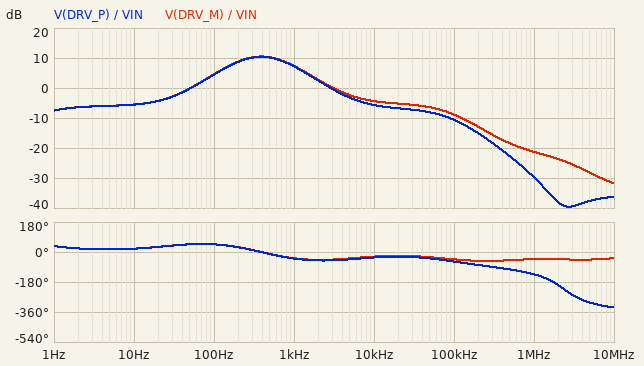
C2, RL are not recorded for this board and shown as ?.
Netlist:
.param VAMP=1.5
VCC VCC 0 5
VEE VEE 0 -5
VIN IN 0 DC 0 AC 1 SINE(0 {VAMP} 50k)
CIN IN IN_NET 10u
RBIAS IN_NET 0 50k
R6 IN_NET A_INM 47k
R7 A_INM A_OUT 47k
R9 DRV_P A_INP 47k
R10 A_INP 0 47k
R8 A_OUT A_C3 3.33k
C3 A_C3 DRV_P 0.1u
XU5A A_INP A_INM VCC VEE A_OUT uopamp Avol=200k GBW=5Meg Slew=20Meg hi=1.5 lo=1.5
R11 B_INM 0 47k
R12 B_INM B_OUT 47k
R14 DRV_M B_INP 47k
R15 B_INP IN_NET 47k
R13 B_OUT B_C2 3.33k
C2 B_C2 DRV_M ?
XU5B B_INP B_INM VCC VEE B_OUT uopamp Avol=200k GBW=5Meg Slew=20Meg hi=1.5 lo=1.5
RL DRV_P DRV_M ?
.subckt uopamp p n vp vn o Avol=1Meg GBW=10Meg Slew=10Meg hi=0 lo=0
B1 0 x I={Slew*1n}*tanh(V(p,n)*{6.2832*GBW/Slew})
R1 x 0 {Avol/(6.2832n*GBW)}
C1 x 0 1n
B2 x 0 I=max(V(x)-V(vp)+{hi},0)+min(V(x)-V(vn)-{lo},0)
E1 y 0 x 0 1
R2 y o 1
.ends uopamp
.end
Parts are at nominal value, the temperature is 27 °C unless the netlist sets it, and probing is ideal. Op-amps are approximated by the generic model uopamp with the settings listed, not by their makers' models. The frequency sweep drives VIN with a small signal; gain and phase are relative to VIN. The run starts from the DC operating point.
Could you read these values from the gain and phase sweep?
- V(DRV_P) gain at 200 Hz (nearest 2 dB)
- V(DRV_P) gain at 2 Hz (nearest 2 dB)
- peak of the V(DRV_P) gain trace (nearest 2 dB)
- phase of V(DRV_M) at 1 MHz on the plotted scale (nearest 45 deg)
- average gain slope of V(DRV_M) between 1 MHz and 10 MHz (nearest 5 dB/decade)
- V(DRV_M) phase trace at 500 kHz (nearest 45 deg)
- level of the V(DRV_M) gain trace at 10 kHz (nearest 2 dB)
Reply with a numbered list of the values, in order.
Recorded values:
1. 8 dB
2. -6 dB
3. 10 dB
4. -45 deg
5. -10 dB/decade
6. -45 deg
7. -4 dB
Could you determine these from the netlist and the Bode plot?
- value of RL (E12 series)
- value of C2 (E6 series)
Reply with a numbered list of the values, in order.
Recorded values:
1. 330 Ω
2. 150 nF
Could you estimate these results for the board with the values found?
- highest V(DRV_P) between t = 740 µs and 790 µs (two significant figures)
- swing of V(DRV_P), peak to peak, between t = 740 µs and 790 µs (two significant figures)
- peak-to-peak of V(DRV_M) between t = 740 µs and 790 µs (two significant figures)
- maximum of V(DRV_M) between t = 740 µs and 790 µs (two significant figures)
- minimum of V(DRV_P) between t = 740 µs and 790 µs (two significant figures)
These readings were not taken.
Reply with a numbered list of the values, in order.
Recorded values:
1. 580 mV
2. 1.2 V
3. 1.4 V
4. 710 mV
5. -600 mV
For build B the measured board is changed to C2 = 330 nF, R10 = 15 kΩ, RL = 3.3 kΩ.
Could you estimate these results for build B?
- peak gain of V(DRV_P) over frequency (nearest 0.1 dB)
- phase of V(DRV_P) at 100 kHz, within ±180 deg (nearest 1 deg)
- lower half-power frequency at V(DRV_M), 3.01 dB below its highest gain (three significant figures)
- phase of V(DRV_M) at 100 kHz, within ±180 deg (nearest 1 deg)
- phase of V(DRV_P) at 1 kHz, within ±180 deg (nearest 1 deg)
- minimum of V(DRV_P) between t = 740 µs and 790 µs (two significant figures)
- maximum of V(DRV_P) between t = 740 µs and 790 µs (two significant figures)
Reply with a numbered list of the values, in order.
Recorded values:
1. 8.4 dB
2. -101 deg
3. 39.2 Hz
4. -8 deg
5. -78 deg
6. -57 mV
7. 68 mV
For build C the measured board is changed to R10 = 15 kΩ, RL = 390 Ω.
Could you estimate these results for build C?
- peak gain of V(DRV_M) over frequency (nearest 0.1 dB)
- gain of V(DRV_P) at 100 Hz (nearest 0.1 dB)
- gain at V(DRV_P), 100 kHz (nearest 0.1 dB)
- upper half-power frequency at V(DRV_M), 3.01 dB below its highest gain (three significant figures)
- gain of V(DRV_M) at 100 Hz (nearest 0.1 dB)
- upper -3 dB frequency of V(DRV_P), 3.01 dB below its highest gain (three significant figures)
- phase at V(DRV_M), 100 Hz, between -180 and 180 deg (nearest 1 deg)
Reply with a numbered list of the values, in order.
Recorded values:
1. -1.8 dB
2. -2.2 dB
3. -25.8 dB
4. 446 Hz
5. -2.0 dB
6. 429 Hz
7. 5 deg
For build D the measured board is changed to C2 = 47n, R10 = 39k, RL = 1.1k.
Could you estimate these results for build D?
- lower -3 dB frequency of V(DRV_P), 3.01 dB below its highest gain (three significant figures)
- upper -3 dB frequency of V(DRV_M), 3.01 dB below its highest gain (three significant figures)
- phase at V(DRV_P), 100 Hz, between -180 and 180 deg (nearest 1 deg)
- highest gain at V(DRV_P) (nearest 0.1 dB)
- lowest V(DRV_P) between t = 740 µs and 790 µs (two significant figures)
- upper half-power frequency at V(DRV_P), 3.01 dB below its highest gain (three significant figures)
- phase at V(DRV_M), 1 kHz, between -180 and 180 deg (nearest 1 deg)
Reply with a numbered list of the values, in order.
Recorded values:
1. 151 Hz
2. 1.44 kHz
3. -102 deg
4. 7.6 dB
5. -200 mV
6. 1.38 kHz
7. 140 deg
